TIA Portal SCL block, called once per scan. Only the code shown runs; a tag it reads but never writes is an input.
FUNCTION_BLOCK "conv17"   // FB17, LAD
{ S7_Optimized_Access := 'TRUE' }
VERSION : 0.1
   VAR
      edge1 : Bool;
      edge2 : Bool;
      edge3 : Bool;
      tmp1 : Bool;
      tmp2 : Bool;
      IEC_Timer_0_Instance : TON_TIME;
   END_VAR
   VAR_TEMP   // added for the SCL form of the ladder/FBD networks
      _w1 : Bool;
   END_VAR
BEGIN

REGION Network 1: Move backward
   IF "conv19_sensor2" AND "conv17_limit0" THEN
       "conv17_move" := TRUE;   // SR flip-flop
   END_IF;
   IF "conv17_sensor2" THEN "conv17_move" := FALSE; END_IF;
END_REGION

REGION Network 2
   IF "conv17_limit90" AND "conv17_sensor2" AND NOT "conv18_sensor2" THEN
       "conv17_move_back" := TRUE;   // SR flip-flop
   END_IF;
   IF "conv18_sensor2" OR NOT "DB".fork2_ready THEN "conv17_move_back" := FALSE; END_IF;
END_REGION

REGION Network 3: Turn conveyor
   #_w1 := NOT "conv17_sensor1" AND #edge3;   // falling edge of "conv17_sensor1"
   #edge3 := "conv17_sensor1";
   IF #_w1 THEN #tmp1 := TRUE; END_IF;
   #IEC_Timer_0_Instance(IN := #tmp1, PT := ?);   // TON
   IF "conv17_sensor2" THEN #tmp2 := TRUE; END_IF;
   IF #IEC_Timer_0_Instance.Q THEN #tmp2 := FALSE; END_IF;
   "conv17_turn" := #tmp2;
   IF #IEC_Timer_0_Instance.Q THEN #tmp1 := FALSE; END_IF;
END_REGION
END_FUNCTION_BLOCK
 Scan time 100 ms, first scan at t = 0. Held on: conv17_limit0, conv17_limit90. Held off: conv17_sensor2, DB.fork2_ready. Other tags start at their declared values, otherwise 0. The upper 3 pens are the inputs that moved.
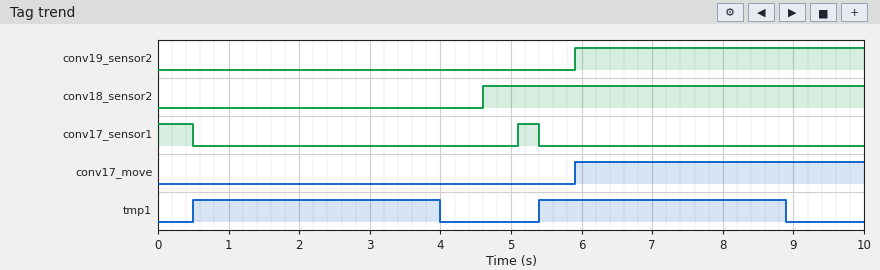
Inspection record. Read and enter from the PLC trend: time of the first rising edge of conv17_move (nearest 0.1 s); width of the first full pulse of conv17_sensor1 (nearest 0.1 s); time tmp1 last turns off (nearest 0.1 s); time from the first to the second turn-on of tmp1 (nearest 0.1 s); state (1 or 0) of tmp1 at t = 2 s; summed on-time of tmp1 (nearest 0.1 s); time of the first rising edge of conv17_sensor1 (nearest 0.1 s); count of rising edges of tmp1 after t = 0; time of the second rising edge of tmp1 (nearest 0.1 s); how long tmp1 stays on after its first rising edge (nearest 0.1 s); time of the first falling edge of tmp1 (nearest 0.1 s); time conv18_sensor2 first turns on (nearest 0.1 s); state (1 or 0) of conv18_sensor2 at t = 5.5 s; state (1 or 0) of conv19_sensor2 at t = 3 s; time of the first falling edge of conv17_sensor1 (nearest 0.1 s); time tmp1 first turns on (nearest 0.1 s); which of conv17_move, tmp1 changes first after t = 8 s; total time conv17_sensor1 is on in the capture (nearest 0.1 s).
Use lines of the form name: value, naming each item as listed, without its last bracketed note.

time of the first rising edge of conv17_move: 5.9 s
width of the first full pulse of conv17_sensor1: 0.3 s
time tmp1 last turns off: 8.9 s
time from the first to the second turn-on of tmp1: 4.9 s
state (1 or 0) of tmp1 at t = 2 s: 1
summed on-time of tmp1: 7.0 s
time of the first rising edge of conv17_sensor1: 5.1 s
count of rising edges of tmp1 after t = 0: 2
time of the second rising edge of tmp1: 5.4 s
how long tmp1 stays on after its first rising edge: 3.5 s
time of the first falling edge of tmp1: 4.0 s
time conv18_sensor2 first turns on: 4.6 s
state (1 or 0) of conv18_sensor2 at t = 5.5 s: 1
state (1 or 0) of conv19_sensor2 at t = 3 s: 0
time of the first falling edge of conv17_sensor1: 0.5 s
time tmp1 first turns on: 0.5 s
which of conv17_move, tmp1 changes first after t = 8 s: tmp1
total time conv17_sensor1 is on in the capture: 0.8 s
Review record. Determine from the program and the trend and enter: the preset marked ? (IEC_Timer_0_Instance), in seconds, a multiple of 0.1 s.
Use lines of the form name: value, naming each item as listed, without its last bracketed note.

the preset marked ? (IEC_Timer_0_Instance), in seconds, a multiple of 0.1 s: 3.5 s
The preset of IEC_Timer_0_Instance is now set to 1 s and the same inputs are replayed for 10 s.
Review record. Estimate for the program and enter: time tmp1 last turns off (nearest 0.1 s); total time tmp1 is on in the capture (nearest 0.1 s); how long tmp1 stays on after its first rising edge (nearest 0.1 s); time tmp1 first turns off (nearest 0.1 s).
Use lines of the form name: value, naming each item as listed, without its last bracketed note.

time tmp1 last turns off: 6.4 s
total time tmp1 is on in the capture: 2.0 s
how long tmp1 stays on after its first rising edge: 1.0 s
time tmp1 first turns off: 1.5 s
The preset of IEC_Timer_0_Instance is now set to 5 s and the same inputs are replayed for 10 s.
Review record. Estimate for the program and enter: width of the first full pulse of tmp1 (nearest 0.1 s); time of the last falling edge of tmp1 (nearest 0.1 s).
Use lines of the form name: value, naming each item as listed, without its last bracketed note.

width of the first full pulse of tmp1: 5.0 s
time of the last falling edge of tmp1: 5.5 s
